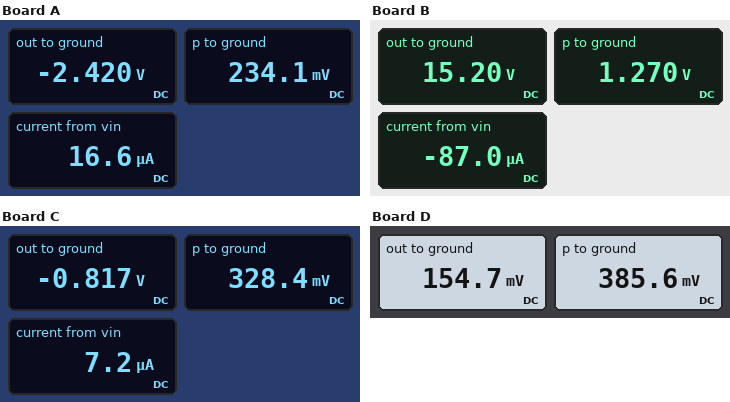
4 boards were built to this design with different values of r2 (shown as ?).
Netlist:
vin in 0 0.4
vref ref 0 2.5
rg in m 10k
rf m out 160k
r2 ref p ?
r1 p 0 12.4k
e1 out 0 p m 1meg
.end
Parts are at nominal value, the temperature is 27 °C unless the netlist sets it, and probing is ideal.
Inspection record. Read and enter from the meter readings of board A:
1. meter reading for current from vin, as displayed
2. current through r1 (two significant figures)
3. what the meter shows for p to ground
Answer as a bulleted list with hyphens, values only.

- 16.6 µA
- 19 µA
- 234.1 mV
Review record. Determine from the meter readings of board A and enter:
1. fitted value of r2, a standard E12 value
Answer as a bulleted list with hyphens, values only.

- 120 kΩ
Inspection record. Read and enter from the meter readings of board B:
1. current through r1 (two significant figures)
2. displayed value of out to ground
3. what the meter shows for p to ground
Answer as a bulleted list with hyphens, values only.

- 100 µA
- 15.20 V
- 1.270 V
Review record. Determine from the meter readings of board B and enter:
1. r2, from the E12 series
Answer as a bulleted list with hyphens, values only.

- 12 kΩ
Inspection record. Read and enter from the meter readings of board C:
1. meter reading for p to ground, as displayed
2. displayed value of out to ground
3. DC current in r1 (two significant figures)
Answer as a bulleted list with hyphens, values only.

- 328.4 mV
- -0.817 V
- 26 µA
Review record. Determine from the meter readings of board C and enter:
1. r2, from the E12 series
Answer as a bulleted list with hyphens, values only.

- 82 kΩ
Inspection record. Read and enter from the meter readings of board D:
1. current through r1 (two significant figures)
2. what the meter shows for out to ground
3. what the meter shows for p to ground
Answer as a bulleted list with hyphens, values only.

- 31 µA
- 154.7 mV
- 385.6 mV
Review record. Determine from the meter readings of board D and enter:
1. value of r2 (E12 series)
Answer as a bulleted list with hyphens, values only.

- 68 kΩ
